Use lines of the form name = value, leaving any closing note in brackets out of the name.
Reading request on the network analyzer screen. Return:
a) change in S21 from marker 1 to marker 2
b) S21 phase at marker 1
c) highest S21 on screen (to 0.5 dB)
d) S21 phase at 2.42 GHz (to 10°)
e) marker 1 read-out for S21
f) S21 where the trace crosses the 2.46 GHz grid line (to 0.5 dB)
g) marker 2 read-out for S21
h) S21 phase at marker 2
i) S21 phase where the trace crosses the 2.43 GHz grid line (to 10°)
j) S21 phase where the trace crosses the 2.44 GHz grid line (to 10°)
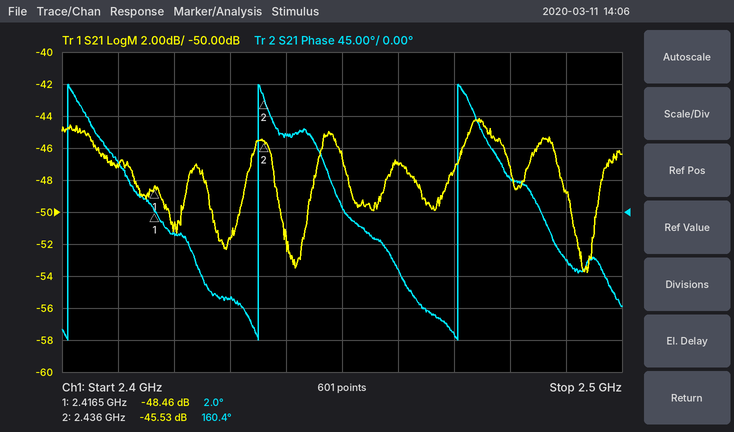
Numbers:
change in S21 from marker 1 to marker 2 = 2.93 dB
S21 phase at marker 1 = 2.0°
highest S21 on screen = -44.0 dB
S21 phase at 2.42 GHz = -30°
marker 1 read-out for S21 = -48.46 dB
S21 where the trace crosses the 2.46 GHz grid line = -47.0 dB
marker 2 read-out for S21 = -45.53 dB
S21 phase at marker 2 = 160.4°
S21 phase where the trace crosses the 2.43 GHz grid line = -120°
S21 phase where the trace crosses the 2.44 GHz grid line = 110°
